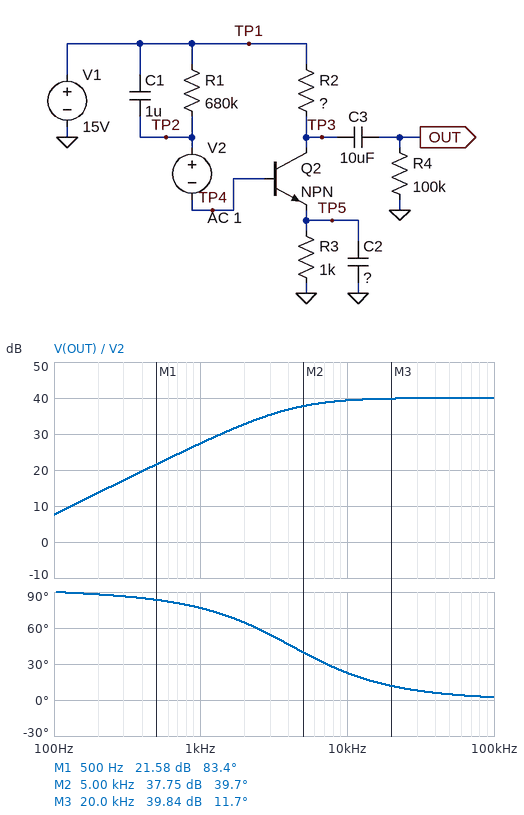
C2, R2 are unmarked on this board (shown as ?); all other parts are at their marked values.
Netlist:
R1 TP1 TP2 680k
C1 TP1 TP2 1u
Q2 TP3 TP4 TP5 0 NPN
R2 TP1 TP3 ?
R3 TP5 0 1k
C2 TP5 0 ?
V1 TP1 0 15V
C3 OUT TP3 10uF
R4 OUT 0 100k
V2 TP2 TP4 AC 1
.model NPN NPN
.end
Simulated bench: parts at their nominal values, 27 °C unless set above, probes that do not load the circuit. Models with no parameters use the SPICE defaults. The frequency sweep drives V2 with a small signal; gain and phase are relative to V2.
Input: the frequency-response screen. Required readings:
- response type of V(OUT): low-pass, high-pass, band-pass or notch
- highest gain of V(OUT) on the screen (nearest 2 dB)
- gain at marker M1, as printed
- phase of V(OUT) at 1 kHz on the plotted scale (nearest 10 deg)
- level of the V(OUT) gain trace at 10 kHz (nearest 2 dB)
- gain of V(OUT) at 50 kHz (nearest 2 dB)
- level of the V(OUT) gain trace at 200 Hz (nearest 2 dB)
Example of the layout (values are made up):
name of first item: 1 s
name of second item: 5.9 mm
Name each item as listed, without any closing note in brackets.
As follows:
response type of V(OUT): low-pass, high-pass, band-pass or notch: high-pass
highest gain of V(OUT) on the screen: 40 dB
gain at marker M1, as printed: 21.58 dB
phase of V(OUT) at 1 kHz on the plotted scale: 80 deg
level of the V(OUT) gain trace at 10 kHz: 40 dB
gain of V(OUT) at 50 kHz: 40 dB
level of the V(OUT) gain trace at 200 Hz: 14 dB
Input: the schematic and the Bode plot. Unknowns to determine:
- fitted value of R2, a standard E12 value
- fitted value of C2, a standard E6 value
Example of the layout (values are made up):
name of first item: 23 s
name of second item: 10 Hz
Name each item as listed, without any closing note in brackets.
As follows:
fitted value of R2, a standard E12 value: 10 kΩ
fitted value of C2, a standard E6 value: 6.8 µF
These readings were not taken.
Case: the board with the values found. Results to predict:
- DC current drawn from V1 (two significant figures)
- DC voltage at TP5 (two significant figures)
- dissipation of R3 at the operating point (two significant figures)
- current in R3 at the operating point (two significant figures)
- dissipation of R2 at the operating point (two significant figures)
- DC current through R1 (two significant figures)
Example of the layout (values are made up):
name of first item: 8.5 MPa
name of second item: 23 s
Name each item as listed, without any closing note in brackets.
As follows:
DC current drawn from V1: 1.4 mA
DC voltage at TP5: 1.4 V
dissipation of R3 at the operating point: 1.9 mW
current in R3 at the operating point: 1.4 mA
dissipation of R2 at the operating point: 18 mW
DC current through R1: 19 µA
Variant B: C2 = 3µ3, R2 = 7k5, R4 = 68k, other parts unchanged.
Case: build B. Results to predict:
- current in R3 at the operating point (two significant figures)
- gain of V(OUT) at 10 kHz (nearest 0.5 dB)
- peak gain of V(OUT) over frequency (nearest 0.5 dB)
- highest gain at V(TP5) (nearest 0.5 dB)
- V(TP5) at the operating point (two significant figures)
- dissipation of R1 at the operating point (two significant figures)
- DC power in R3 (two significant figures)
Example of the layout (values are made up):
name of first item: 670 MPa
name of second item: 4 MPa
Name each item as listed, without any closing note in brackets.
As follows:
current in R3 at the operating point: 1.8 mA
gain of V(OUT) at 10 kHz: 49.0 dB
peak gain of V(OUT) over frequency: 50.0 dB
highest gain at V(TP5): -4.5 dB
V(TP5) at the operating point: 1.8 V
dissipation of R1 at the operating point: 230 µW
DC power in R3: 3.1 mW
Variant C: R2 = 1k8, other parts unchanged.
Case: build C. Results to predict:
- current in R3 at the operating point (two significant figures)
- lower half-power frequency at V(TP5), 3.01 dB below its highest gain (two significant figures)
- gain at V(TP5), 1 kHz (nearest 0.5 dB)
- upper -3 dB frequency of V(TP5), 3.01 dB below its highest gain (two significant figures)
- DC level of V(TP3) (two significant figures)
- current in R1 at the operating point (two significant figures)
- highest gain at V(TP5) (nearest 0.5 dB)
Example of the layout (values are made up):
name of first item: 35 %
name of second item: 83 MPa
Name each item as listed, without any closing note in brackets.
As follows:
current in R3 at the operating point: 1.8 mA
lower half-power frequency at V(TP5), 3.01 dB below its highest gain: 1.6 Hz
gain at V(TP5), 1 kHz: -2.0 dB
upper -3 dB frequency of V(TP5), 3.01 dB below its highest gain: 1.8 kHz
DC level of V(TP3): 12 V
current in R1 at the operating point: 18 µA
highest gain at V(TP5): -0.5 dB
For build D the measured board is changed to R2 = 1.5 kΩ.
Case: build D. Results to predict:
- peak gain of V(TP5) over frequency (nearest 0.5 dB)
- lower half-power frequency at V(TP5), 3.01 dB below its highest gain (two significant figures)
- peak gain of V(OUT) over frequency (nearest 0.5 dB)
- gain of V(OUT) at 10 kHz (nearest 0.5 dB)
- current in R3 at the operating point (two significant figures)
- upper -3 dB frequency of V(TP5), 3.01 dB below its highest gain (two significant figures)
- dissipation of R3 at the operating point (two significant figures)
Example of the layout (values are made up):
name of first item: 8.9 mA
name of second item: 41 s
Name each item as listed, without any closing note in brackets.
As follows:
peak gain of V(TP5) over frequency: -0.5 dB
lower half-power frequency at V(TP5), 3.01 dB below its highest gain: 1.6 Hz
peak gain of V(OUT) over frequency: 40.5 dB
gain of V(OUT) at 10 kHz: 40.0 dB
current in R3 at the operating point: 1.8 mA
upper -3 dB frequency of V(TP5), 3.01 dB below its highest gain: 1.8 kHz
dissipation of R3 at the operating point: 3.4 mW
